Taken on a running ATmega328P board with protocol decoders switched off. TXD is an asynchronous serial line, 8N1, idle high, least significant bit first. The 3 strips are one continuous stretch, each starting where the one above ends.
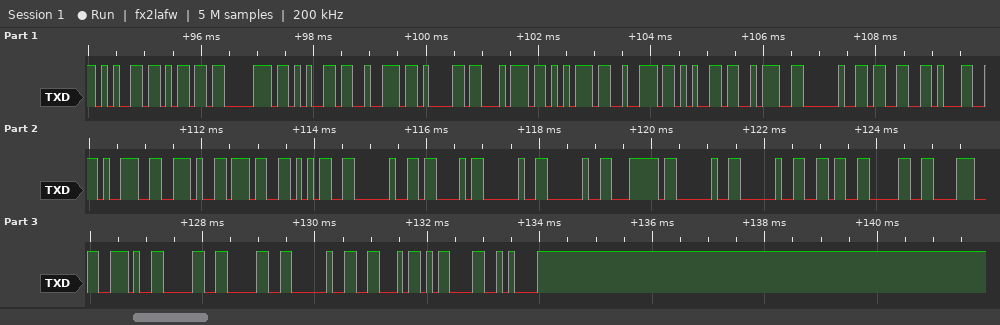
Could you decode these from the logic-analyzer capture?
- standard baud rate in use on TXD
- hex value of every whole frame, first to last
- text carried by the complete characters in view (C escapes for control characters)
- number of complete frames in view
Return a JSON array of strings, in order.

["9600 baud", "65 6D 70 65 72 61 74 75 72 65 3A 20 33 31 39 2E 37 35 20 43 20 20 7C 20 20 36 30 38 2E 30 30 20 46 0D 0A", "\"emperature: 319.75 C  |  608.00 F\\r\\n\"", "35"]
